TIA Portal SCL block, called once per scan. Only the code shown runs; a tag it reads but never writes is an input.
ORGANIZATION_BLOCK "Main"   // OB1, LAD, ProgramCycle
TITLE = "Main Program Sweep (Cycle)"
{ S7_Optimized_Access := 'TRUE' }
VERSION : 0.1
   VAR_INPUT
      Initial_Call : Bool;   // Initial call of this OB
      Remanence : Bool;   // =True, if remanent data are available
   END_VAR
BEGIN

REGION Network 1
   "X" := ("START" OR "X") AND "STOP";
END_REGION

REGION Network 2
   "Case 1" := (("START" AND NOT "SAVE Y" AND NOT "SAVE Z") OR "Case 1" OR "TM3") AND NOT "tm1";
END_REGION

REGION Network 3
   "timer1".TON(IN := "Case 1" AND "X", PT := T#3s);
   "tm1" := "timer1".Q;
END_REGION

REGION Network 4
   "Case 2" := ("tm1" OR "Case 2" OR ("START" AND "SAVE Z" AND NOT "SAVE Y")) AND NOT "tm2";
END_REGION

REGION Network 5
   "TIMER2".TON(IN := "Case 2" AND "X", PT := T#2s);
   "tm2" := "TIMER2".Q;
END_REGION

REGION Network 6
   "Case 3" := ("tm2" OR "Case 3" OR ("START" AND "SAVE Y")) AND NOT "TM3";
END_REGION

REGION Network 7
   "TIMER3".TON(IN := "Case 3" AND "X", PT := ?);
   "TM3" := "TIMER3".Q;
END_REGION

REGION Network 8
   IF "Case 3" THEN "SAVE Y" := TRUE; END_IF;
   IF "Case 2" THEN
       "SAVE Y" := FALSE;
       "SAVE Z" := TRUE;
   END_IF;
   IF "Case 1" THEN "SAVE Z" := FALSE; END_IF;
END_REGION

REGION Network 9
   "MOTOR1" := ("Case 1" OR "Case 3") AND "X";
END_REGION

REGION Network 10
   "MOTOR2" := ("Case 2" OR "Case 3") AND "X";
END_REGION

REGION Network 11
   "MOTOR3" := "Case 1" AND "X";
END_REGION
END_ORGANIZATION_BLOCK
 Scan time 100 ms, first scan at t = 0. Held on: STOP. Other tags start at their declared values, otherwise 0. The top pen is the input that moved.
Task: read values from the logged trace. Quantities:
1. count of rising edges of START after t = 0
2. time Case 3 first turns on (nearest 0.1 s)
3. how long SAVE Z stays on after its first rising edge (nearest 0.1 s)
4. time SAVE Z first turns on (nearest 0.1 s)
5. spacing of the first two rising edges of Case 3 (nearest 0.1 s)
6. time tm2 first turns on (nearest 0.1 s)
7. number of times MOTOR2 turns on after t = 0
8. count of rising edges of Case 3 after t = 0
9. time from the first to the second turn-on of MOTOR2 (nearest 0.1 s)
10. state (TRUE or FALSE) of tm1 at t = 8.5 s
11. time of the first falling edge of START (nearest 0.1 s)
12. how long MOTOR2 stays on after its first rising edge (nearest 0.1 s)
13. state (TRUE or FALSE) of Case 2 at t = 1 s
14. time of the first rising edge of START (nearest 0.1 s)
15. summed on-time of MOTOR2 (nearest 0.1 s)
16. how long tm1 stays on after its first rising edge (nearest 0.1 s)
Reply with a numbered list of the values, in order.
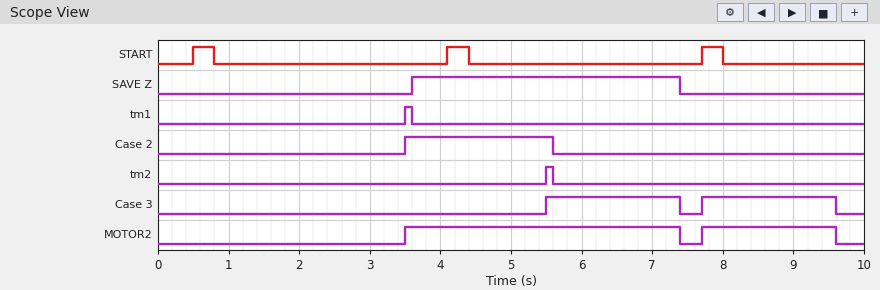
1. 3
2. 5.5 s
3. 3.8 s
4. 3.6 s
5. 2.2 s
6. 5.5 s
7. 2
8. 2
9. 4.2 s
10. FALSE
11. 0.8 s
12. 3.9 s
13. FALSE
14. 0.5 s
15. 5.8 s
16. 0.1 s
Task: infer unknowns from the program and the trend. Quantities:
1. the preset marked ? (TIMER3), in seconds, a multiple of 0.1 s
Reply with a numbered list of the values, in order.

1. 1.8 s
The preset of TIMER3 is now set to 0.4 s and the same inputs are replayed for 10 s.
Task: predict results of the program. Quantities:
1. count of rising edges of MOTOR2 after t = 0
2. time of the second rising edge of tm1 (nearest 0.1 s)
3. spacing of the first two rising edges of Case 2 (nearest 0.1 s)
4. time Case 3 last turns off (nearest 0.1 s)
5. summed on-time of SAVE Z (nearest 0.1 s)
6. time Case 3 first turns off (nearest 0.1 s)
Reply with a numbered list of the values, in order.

1. 3
2. 9.0 s
3. 5.5 s
4. 8.2 s
5. 3.3 s
6. 6.0 s
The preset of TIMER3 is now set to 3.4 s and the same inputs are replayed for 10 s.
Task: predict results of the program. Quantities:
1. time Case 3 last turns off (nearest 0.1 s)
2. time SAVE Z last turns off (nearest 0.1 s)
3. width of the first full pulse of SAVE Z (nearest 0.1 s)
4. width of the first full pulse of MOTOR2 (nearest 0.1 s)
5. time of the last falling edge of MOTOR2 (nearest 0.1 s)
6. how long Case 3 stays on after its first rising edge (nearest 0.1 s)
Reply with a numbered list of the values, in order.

1. 9.0 s
2. 9.0 s
3. 5.4 s
4. 5.5 s
5. 9.0 s
6. 3.5 s
